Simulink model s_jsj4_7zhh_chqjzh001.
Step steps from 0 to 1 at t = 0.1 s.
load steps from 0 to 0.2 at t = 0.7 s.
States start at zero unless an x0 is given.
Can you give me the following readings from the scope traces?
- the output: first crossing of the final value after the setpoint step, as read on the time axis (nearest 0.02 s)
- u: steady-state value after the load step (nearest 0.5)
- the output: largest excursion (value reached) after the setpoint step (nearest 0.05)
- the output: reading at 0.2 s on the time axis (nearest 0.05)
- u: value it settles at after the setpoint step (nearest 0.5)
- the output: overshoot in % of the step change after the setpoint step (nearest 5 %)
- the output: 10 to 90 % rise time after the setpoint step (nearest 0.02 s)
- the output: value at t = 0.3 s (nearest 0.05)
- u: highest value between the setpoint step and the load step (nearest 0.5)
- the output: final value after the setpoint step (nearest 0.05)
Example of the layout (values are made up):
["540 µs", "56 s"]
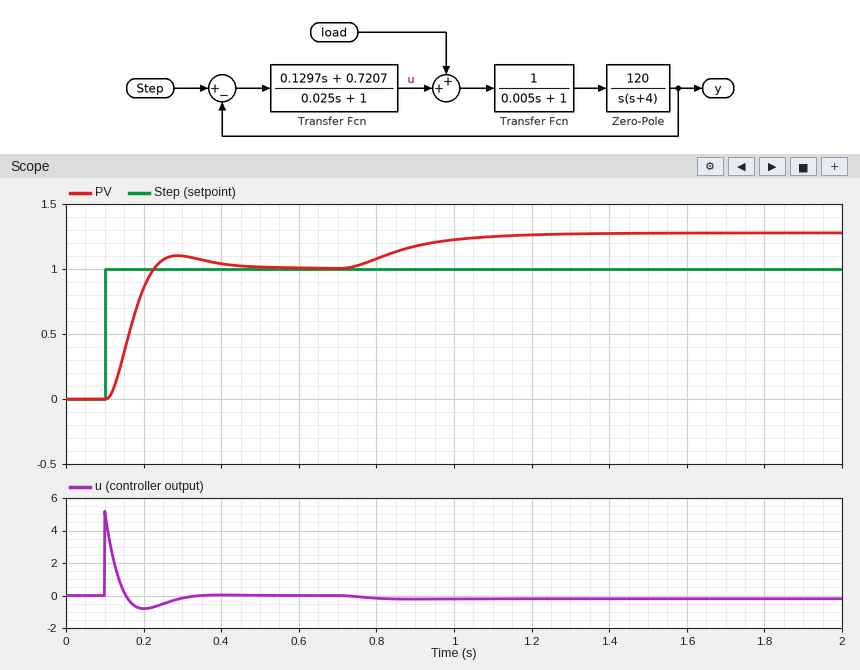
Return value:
["0.22 s", "0.0", "1.10", "0.85", "0.0", "10 %", "0.08 s", "1.10", "5.0", "1.00"]
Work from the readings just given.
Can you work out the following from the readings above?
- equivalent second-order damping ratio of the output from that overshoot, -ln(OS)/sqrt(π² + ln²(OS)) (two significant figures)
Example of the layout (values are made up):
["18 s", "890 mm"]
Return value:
["0.59"]
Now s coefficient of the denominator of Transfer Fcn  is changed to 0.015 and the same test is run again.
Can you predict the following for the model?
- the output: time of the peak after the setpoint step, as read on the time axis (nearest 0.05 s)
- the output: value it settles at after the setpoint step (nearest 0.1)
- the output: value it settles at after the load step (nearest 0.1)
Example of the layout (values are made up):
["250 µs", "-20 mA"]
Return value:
["0.30 s", "1.0", "1.3"]
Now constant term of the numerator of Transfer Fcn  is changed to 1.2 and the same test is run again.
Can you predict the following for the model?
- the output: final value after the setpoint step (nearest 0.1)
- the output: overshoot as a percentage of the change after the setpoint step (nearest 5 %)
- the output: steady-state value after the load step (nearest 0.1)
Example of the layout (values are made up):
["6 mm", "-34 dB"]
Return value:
["1.0", "25 %", "1.2"]
